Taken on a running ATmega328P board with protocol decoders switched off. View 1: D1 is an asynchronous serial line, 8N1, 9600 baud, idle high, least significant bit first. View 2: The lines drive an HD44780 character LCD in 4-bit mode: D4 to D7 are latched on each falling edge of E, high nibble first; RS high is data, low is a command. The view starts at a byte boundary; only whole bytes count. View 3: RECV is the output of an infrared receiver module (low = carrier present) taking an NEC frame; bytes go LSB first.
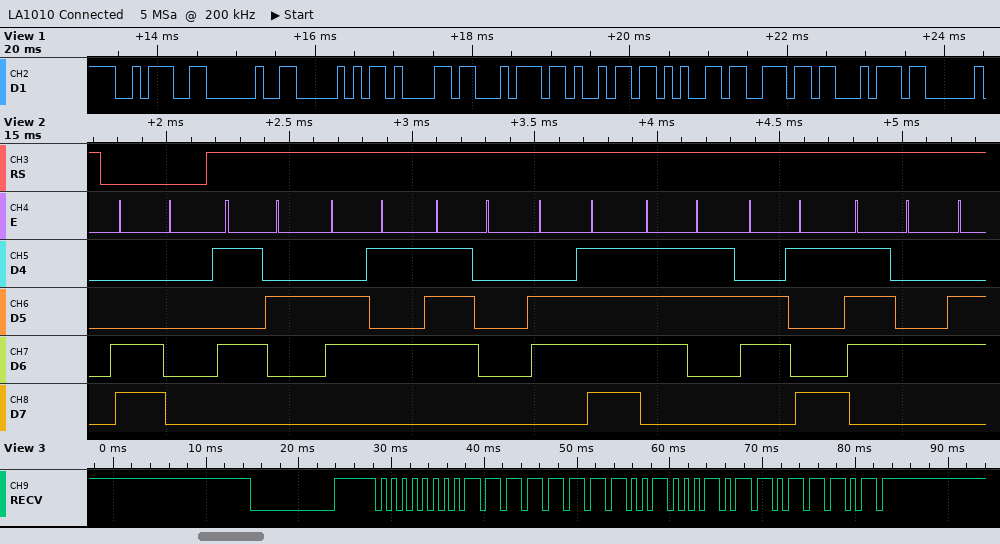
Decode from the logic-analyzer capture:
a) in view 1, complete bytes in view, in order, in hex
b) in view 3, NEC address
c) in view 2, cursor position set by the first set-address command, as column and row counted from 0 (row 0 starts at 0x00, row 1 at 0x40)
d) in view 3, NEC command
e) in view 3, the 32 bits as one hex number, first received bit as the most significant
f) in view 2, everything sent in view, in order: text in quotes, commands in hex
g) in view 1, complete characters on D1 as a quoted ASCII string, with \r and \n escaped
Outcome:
3A 20 50 61 74 69 65 6E 74
0x00
column 0, row 1
0x44
0x00FF22DD
0xC0 "Reposit"
": Patient"
